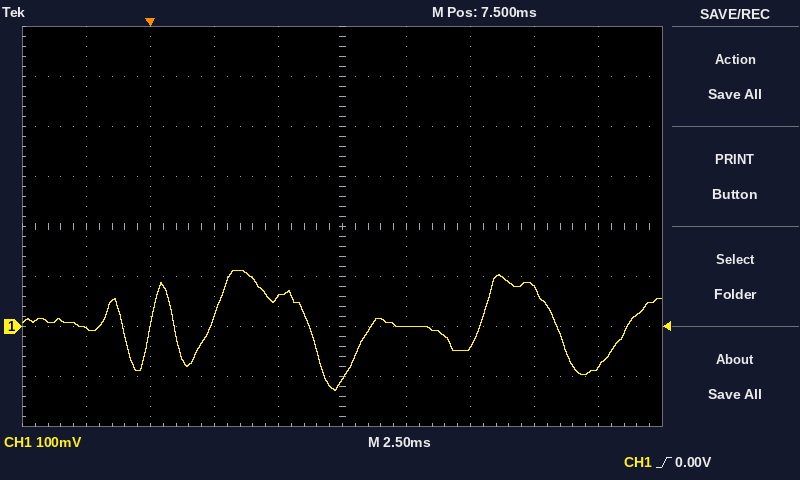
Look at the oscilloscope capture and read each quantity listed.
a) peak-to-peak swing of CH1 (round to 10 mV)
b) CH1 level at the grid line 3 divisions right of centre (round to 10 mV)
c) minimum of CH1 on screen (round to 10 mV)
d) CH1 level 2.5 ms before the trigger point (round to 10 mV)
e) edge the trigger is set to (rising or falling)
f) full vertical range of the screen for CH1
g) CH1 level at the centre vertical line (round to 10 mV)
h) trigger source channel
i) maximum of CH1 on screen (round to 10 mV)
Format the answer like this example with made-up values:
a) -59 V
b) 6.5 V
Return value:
a) 240 mV
b) 80 mV
c) -130 mV
d) 0 mV
e) rising
f) 800 mV
g) -110 mV
h) CH1
i) 110 mV
